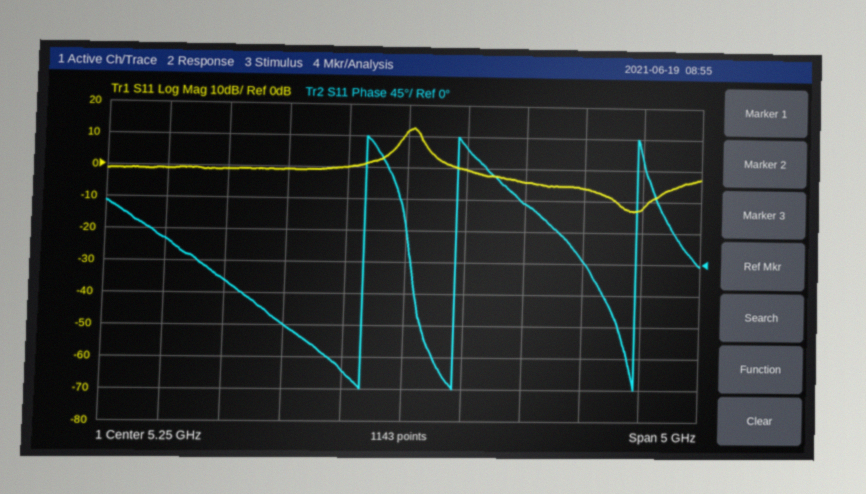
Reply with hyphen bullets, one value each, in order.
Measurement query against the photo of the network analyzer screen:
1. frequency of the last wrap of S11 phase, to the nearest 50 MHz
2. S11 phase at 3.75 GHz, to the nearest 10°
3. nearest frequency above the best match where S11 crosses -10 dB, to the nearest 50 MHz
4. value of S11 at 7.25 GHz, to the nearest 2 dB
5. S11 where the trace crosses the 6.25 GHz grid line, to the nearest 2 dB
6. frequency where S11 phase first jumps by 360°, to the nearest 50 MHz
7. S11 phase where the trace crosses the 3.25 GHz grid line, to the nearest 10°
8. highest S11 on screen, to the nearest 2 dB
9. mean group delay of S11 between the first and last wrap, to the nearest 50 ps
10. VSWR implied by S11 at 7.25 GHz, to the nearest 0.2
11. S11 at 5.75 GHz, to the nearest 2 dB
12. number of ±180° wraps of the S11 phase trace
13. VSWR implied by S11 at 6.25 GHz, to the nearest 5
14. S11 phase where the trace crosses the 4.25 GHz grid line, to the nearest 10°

- 7.20 GHz
- -30°
- 7.30 GHz
- -12 dB
- -4 dB
- 4.90 GHz
- 30°
- 12 dB
- 850 ps
- 1.6
- 0 dB
- 3
- 5
- -90°
